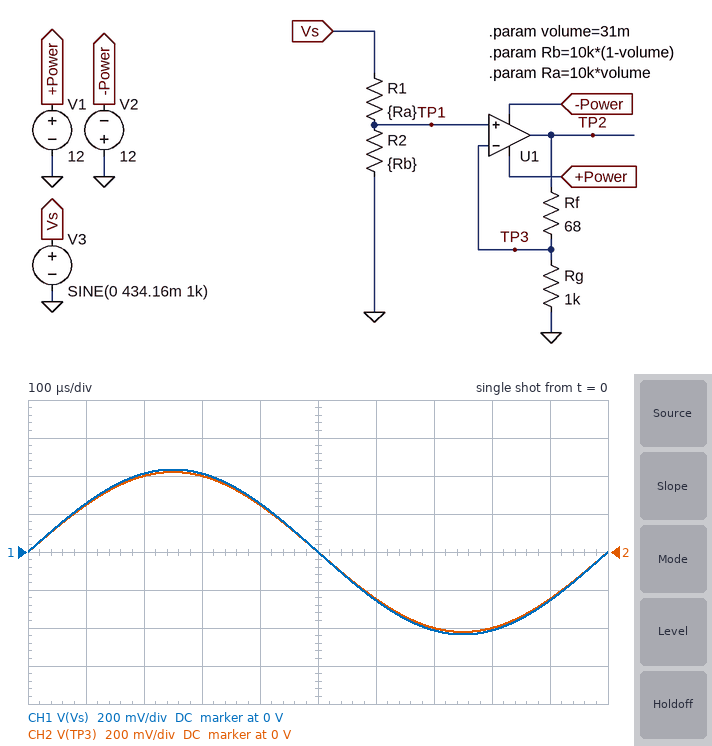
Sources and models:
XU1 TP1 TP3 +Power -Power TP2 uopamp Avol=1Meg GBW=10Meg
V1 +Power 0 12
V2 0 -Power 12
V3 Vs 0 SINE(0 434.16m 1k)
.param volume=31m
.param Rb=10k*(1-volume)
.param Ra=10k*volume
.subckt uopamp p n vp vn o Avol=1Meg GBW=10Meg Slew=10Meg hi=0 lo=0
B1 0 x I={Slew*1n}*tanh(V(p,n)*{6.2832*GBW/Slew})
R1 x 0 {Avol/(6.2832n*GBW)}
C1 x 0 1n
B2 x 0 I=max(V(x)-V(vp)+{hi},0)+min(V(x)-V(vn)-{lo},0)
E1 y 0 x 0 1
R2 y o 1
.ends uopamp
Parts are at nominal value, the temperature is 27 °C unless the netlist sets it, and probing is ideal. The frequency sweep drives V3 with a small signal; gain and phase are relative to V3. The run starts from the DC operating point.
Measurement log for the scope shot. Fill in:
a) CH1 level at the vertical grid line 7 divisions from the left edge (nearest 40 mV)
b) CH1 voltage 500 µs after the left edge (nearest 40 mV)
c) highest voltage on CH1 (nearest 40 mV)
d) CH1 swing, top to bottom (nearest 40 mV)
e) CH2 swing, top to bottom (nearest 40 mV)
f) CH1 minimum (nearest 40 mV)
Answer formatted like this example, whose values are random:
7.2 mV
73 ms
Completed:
-400 mV
0 V
440 mV
880 mV
840 mV
-440 mV
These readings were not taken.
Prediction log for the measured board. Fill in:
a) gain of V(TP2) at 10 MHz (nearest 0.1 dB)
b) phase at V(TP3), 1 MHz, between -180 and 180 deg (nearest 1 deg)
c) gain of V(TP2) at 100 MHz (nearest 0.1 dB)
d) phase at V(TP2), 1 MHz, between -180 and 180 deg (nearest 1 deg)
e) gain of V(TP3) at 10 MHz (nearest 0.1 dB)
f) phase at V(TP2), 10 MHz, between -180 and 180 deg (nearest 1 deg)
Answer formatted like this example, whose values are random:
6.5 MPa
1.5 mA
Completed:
-3.0 dB
-6 deg
-20.3 dB
-6 deg
-3.6 dB
-47 deg
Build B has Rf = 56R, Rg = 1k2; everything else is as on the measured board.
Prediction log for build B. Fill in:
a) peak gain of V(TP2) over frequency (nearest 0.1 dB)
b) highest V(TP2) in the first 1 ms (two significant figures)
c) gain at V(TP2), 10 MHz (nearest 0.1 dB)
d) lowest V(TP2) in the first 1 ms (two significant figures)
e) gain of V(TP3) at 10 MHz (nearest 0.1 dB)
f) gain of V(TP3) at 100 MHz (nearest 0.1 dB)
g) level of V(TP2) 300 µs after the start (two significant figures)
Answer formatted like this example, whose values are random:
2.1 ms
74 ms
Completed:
0.1 dB
440 mV
-3.1 dB
-440 mV
-3.5 dB
-20.7 dB
420 mV
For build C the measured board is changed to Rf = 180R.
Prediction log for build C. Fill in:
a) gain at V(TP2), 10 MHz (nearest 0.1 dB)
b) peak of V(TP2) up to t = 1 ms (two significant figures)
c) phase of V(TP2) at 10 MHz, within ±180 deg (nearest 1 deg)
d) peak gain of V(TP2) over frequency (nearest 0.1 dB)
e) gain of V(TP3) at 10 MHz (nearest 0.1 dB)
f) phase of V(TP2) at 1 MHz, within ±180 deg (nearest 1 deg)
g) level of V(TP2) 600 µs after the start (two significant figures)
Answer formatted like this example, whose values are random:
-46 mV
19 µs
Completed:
-2.6 dB
500 mV
-50 deg
1.2 dB
-4.1 dB
-7 deg
-290 mV
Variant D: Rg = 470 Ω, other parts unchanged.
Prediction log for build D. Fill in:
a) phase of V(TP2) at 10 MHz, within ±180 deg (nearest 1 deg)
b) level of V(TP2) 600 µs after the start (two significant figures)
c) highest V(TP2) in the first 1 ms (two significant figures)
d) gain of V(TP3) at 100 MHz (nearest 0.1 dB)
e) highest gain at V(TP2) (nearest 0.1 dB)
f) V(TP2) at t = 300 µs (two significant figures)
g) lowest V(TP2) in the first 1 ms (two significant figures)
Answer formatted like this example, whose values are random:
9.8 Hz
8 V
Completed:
-49 deg
-280 mV
480 mV
-21.5 dB
0.9 dB
460 mV
-480 mV
